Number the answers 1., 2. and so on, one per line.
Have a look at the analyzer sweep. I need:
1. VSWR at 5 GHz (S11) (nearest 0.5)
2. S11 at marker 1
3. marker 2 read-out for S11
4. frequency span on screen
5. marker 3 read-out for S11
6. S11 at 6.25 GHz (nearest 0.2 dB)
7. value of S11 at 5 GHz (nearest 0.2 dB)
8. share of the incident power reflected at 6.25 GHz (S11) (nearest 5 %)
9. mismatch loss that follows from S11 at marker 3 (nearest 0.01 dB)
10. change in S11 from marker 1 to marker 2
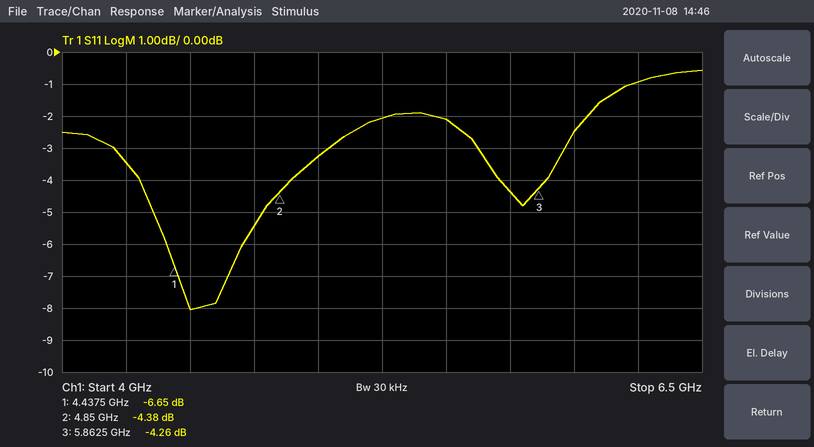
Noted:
1. 5.5
2. -6.65 dB
3. -4.38 dB
4. 2.5 GHz
5. -4.26 dB
6. -1.0 dB
7. -3.2 dB
8. 80 %
9. 2.04 dB
10. 2.27 dB
